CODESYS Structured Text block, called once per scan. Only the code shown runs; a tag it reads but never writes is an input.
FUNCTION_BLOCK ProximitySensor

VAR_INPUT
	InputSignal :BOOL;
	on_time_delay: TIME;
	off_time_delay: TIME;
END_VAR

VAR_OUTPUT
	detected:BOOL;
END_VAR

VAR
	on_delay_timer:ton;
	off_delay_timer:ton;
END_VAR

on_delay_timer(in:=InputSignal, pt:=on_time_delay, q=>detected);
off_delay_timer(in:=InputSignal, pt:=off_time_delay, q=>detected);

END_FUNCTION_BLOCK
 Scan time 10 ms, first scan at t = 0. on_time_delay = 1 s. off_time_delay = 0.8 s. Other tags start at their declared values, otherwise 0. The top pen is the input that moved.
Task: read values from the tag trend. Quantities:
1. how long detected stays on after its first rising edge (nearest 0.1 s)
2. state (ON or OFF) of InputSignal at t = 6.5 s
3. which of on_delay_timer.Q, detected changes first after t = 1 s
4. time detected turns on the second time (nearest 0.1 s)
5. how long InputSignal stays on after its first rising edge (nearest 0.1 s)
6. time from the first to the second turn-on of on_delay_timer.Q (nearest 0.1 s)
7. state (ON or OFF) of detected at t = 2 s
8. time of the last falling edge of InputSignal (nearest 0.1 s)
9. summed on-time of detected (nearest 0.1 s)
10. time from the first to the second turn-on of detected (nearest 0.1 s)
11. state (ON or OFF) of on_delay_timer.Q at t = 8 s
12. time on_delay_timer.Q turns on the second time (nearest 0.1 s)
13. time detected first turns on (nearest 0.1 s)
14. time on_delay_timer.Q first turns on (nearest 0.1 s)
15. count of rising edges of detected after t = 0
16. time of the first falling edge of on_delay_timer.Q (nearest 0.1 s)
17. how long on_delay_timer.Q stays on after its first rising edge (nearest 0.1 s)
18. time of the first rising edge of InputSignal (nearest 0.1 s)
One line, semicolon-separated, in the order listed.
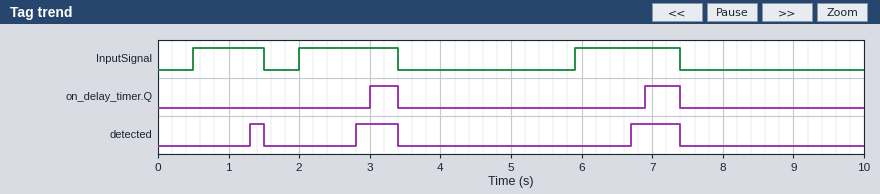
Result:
0.2 s; ON; detected; 2.8 s; 1.0 s; 3.9 s; OFF; 7.4 s; 1.5 s; 1.5 s; OFF; 6.9 s; 1.3 s; 3.0 s; 3; 3.4 s; 0.4 s; 0.5 s
